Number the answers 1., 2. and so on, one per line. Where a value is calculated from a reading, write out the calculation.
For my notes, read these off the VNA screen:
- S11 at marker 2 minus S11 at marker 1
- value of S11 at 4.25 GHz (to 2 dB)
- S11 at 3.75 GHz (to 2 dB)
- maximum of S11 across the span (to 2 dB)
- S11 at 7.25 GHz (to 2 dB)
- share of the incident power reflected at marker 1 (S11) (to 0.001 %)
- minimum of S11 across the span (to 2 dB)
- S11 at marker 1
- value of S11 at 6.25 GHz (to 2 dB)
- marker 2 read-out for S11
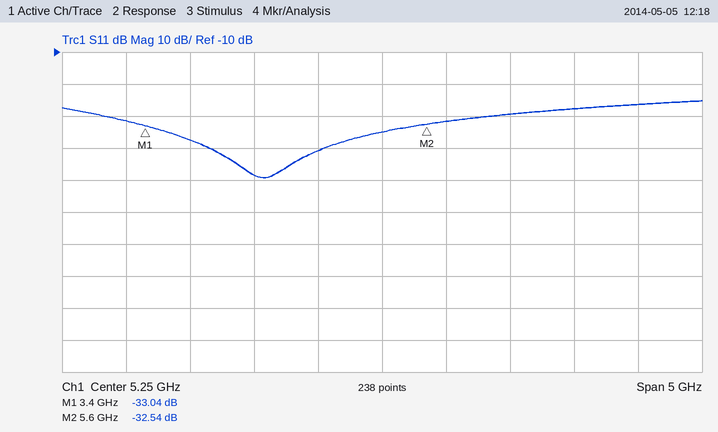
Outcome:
1. -32.54 − (-33.04) = 0.50 dB
2. -48 dB
3. -38 dB
4. -26 dB
5. -26 dB
6. 10^(-33.04/10) ≈ 0.050 %
7. -50 dB
8. -33.04 dB
9. -30 dB
10. -32.54 dB
